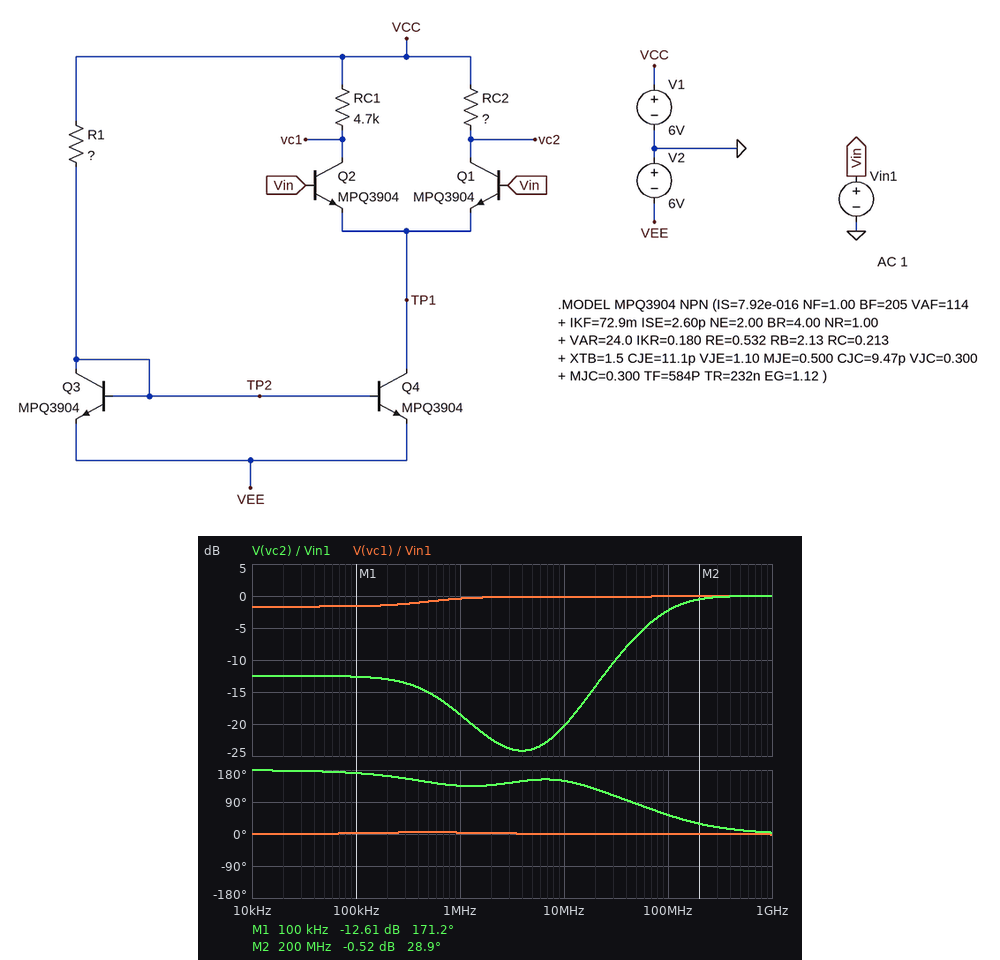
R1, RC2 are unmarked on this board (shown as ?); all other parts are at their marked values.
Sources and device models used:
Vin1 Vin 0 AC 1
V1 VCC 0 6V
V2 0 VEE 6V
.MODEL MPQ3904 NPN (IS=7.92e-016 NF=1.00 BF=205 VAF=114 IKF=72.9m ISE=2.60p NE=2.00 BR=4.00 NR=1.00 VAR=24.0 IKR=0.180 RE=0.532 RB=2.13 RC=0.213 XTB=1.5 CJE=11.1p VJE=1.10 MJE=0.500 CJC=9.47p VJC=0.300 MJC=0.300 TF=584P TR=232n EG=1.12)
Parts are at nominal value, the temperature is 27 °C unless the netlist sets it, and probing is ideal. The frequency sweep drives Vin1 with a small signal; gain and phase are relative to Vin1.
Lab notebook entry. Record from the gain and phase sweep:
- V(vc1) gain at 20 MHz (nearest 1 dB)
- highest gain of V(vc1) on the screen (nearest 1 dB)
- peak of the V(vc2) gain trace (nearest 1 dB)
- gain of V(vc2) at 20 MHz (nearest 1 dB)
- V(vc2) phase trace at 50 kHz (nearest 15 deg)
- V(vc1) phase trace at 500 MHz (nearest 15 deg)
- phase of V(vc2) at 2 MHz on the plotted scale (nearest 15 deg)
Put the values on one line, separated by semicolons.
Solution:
0 dB; 0 dB; 0 dB; -14 dB; 180 deg; 0 deg; 135 deg
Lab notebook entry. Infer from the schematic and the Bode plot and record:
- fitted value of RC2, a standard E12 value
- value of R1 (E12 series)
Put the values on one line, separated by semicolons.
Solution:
1.8 kΩ; 3.9 kΩ
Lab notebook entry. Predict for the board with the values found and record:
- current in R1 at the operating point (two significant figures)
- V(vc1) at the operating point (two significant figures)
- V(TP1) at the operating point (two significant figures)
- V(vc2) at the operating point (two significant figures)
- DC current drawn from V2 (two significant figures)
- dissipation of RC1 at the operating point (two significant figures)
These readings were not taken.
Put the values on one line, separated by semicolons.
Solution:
2.9 mA; -640 mV; -730 mV; 3.3 V; 5.8 mA; 9.4 mW
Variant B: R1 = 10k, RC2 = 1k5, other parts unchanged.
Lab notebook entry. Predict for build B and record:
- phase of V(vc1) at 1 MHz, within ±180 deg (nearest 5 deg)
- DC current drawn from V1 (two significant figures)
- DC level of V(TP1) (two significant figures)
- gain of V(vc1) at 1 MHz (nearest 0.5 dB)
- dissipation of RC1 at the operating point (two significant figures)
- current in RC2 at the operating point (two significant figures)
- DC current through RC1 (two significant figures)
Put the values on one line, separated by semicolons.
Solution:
155 deg; 2.3 mA; -710 mV; -32.0 dB; 1.5 mW; 580 µA; 570 µA
